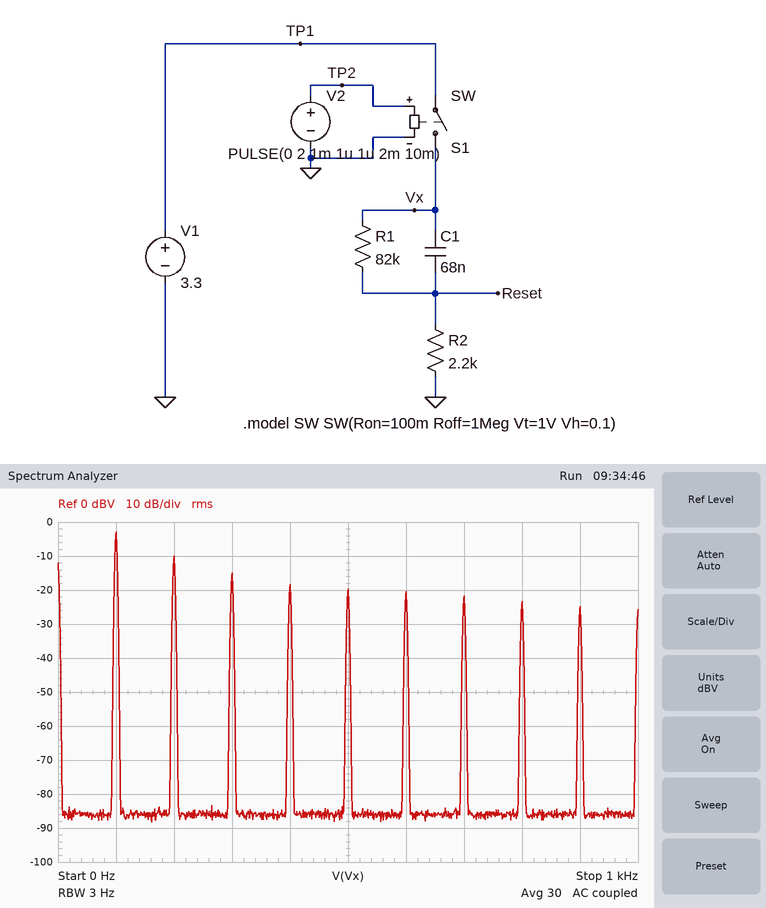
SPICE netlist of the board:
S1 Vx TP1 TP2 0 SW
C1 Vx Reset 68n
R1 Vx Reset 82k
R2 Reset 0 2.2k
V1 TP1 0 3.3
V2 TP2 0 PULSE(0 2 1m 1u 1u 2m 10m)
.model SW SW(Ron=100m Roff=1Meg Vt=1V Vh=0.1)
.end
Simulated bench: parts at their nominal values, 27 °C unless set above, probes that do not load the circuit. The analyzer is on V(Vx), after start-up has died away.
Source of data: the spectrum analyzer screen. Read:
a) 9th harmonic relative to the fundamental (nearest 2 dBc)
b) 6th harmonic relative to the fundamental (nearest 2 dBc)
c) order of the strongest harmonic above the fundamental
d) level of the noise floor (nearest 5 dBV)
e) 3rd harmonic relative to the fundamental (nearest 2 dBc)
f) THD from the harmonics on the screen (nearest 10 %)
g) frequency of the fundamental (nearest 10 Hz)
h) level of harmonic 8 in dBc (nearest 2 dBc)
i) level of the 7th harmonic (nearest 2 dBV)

-22 dBc
-18 dBc
2
-85 dBV
-12 dBc
60 %
100 Hz
-20 dBc
-22 dBV
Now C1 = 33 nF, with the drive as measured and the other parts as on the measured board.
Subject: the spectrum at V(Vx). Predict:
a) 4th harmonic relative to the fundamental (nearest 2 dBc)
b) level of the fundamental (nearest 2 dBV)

-16 dBc
0 dBV
